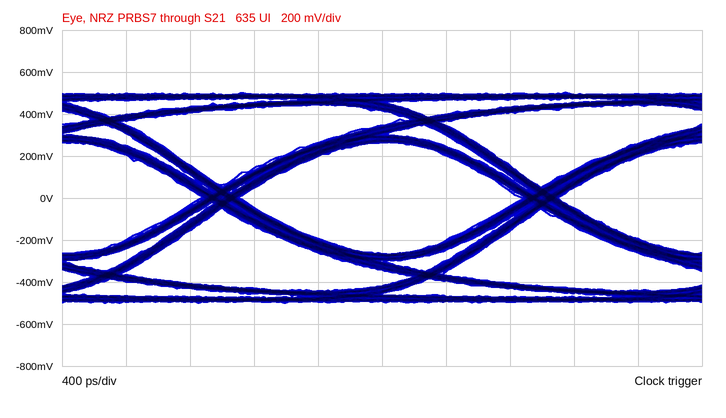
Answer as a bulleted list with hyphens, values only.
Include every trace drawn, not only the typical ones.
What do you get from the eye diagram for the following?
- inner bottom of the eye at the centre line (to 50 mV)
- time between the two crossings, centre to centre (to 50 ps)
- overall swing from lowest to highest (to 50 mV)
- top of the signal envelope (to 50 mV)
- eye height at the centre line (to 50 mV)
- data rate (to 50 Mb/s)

- -250 mV
- 2.00 ns
- 1.00 V
- 500 mV
- 550 mV
- 500 Mb/s
